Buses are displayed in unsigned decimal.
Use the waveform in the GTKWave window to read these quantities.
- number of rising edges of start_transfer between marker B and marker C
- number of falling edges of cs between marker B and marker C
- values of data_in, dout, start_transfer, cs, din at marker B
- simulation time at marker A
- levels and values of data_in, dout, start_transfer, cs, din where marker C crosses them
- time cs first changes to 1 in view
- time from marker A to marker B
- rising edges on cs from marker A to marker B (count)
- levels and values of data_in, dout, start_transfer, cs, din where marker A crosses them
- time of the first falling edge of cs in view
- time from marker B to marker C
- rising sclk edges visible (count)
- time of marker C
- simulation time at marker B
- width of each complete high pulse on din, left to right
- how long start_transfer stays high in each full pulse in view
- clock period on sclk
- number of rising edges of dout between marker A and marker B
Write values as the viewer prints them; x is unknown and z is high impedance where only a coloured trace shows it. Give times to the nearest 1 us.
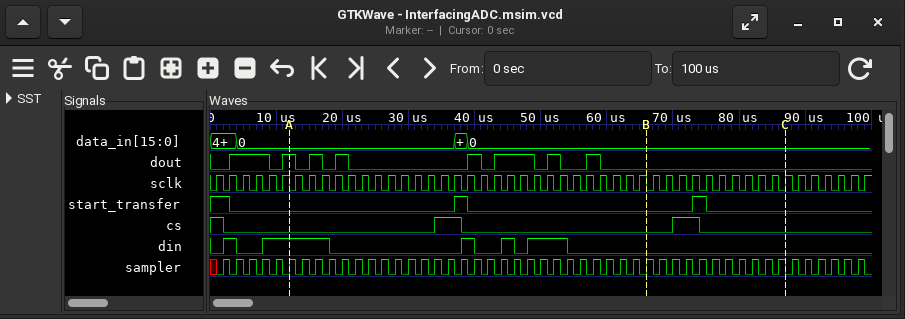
1
1
data_in=0, dout=0, start_transfer=0, cs=0, din=0
12 us
data_in=0, dout=0, start_transfer=0, cs=0, din=0
34 us
54 us
1
data_in=0, dout=1, start_transfer=0, cs=0, din=1
2 us
21 us
50
87 us
66 us
2 us, 10 us, 2 us, 2 us, 6 us
2 us, 2 us
2 us
6
